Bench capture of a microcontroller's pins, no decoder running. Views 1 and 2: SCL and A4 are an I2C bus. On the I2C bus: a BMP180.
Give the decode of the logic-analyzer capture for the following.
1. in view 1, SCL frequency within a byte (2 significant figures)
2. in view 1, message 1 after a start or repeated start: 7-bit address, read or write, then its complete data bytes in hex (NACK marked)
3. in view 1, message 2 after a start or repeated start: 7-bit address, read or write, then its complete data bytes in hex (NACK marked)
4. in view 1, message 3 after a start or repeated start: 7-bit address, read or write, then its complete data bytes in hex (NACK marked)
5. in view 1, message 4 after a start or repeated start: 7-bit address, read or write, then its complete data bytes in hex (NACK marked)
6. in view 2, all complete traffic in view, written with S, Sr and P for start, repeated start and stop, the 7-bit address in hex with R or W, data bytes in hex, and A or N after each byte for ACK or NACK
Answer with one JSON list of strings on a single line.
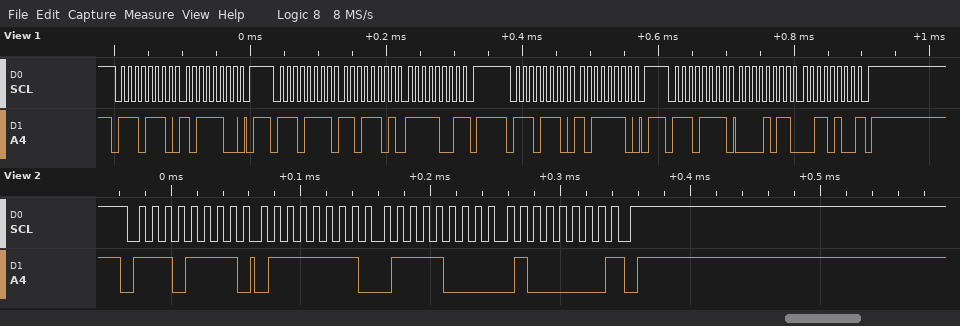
["100 kHz", "0x77 write: BC", "0x77 read: DD F9 NACK", "0x77 write: BE", "0x77 read: 0B 34 NACK", "S 77R A 7F A 78 A 40 N P"]
